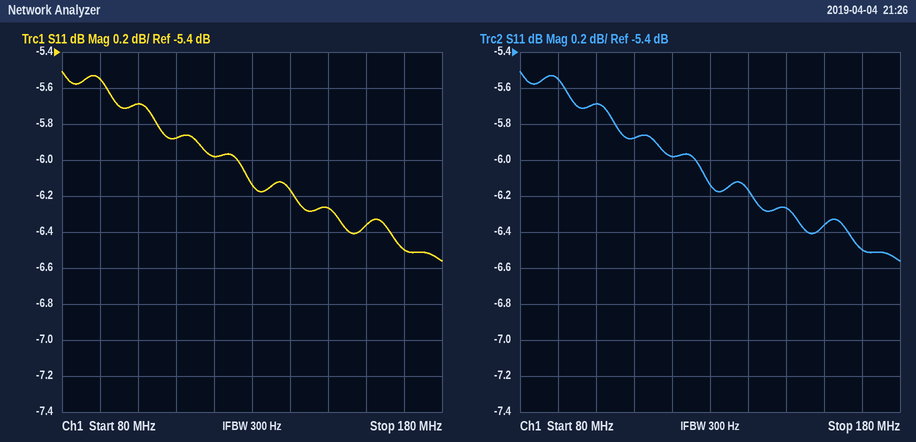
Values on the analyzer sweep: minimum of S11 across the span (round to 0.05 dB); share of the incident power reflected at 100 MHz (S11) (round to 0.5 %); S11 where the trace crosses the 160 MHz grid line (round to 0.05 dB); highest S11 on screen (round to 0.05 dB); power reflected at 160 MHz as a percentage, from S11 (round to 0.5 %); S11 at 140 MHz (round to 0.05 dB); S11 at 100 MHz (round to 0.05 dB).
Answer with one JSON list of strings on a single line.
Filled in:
["-6.55 dB", "27.0 %", "-6.35 dB", "-5.50 dB", "23.0 %", "-6.15 dB", "-5.70 dB"]
